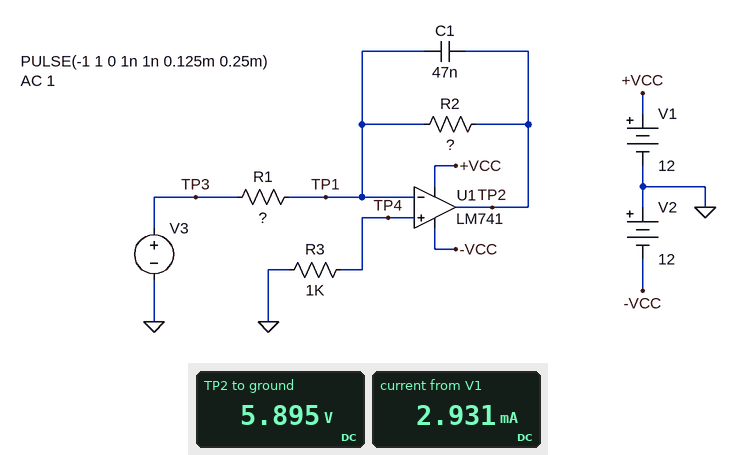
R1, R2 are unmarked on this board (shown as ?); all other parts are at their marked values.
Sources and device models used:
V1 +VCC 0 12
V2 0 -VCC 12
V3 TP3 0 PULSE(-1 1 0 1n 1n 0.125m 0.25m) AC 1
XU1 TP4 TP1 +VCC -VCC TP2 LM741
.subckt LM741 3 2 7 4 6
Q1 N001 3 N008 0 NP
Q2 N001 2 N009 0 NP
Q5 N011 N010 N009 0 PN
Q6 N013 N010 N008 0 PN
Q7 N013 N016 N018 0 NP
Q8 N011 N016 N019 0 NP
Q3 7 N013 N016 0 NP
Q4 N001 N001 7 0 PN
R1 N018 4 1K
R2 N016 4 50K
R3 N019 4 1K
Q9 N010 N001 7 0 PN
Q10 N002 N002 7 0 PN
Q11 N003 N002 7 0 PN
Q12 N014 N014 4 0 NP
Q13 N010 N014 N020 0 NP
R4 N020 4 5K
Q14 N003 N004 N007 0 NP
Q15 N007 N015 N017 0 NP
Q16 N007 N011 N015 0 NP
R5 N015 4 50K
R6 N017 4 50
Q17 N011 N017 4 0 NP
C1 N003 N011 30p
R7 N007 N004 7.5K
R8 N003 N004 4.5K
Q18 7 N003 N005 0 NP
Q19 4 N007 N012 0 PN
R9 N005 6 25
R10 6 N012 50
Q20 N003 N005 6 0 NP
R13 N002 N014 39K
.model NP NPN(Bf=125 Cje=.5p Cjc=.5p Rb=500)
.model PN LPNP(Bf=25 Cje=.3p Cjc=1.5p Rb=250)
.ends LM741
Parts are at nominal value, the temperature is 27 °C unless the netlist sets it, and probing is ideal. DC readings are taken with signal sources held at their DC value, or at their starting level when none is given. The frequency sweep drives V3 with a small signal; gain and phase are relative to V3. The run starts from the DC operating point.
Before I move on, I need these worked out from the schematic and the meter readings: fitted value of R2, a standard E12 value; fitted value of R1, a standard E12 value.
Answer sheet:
3.3 kΩ
560 Ω
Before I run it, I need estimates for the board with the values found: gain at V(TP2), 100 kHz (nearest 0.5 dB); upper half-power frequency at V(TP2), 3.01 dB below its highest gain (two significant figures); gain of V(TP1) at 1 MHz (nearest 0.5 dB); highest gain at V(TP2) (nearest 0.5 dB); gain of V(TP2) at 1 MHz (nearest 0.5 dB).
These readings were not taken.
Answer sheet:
-23.5 dB
1.0 kHz
-25.0 dB
15.5 dB
-24.5 dB
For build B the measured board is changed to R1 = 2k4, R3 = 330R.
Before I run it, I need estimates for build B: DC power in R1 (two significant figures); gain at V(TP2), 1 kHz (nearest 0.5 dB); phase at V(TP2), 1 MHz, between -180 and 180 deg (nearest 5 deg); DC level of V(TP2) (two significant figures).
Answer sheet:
420 µW
0 dB
45 deg
1.4 V
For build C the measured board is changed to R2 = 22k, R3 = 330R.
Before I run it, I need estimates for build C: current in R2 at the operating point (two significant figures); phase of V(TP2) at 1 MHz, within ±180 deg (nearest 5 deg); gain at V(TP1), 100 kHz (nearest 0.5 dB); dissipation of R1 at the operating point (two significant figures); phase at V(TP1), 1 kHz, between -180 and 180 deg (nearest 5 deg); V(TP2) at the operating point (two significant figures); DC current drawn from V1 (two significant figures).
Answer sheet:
540 µA
0 deg
-17.5 dB
160 µW
-10 deg
11 V
1.2 mA
